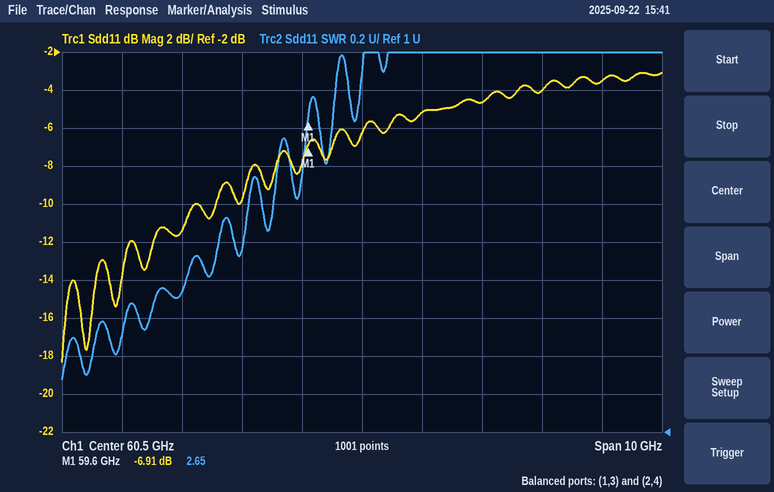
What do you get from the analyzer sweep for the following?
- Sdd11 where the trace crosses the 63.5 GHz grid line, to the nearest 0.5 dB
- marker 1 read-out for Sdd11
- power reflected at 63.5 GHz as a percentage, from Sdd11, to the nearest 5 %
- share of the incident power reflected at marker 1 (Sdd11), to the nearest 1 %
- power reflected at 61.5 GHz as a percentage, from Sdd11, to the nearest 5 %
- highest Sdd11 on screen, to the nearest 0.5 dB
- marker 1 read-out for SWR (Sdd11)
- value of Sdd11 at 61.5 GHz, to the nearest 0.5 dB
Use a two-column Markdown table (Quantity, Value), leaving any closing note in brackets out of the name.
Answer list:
| Quantity | Value |
|---|---|
| Sdd11 where the trace crosses the 63.5 GHz grid line, to the nearest 0.5 dB | -4.0 dB |
| marker 1 read-out for Sdd11 | -6.91 dB |
| power reflected at 63.5 GHz as a percentage, from Sdd11, to the nearest 5 % | 40 % |
| share of the incident power reflected at marker 1 (Sdd11), to the nearest 1 % | 20 % |
| power reflected at 61.5 GHz as a percentage, from Sdd11, to the nearest 5 % | 30 % |
| highest Sdd11 on screen, to the nearest 0.5 dB | -3.0 dB |
| marker 1 read-out for SWR | 2.65 |
| value of Sdd11 at 61.5 GHz, to the nearest 0.5 dB | -5.0 dB |
